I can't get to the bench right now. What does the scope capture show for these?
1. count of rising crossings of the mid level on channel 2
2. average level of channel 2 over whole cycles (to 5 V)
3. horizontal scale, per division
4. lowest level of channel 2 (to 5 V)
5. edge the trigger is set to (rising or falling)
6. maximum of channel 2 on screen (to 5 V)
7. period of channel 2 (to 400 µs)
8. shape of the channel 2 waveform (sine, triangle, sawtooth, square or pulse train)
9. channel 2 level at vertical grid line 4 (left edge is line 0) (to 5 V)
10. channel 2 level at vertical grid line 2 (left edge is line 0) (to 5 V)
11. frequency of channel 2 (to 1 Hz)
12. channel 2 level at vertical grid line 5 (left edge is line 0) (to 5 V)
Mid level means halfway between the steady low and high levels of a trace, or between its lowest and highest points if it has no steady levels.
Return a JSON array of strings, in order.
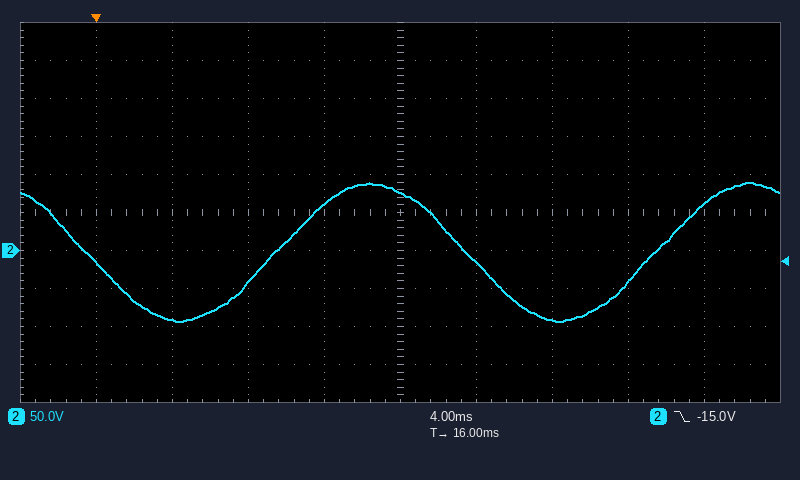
["2", "0 V", "4 ms", "-95 V", "falling", "90 V", "20.0 ms", "sine", "60 V", "-90 V", "50 Hz", "75 V"]
